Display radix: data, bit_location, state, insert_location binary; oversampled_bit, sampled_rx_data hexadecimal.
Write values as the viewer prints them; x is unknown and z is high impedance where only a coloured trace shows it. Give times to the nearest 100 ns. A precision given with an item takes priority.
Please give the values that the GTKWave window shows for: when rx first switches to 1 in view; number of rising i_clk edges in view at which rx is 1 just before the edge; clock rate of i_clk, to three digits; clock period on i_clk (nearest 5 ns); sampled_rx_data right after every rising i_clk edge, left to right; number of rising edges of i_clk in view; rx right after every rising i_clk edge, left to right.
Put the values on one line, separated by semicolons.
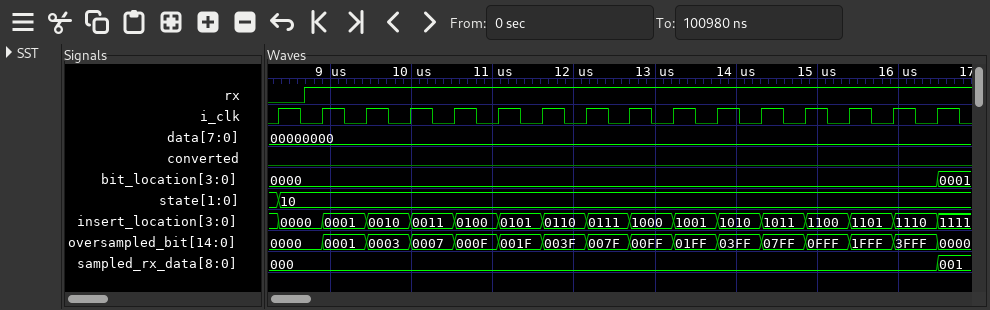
8700 ns; 15; 1.85 MHz; 540 ns; 000, 000, 000, 000, 000, 000, 000, 000, 000, 000, 000, 000, 000, 000, 000, 001; 16; 0 1 1 1 1 1 1 1 1 1 1 1 1 1 1 1
